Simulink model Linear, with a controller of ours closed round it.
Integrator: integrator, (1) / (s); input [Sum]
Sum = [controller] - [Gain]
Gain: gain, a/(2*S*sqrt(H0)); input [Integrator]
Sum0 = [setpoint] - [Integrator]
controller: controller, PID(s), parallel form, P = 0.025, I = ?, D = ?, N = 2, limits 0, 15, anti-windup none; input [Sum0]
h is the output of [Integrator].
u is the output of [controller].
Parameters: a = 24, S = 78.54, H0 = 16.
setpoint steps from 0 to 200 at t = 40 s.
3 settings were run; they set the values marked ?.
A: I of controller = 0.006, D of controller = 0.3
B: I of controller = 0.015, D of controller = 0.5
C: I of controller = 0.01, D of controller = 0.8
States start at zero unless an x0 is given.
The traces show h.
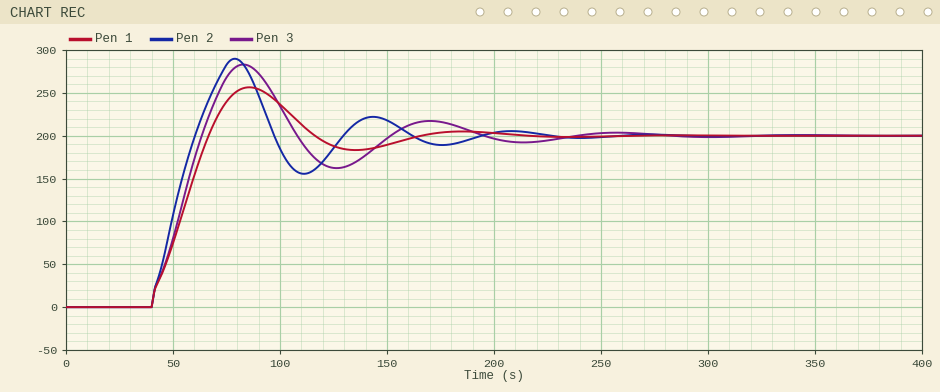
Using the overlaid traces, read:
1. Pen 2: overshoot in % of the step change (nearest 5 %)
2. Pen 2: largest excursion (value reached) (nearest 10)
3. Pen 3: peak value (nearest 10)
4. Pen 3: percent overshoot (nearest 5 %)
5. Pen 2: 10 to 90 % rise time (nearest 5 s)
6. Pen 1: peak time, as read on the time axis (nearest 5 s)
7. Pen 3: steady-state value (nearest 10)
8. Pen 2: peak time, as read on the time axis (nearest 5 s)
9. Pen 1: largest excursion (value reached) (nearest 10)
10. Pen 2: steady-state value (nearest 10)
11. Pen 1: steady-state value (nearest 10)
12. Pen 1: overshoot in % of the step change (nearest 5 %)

45 %
290
280
40 %
15 s
85 s
200
80 s
260
200
200
30 %
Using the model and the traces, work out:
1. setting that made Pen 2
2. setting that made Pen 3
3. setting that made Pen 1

B
C
A
